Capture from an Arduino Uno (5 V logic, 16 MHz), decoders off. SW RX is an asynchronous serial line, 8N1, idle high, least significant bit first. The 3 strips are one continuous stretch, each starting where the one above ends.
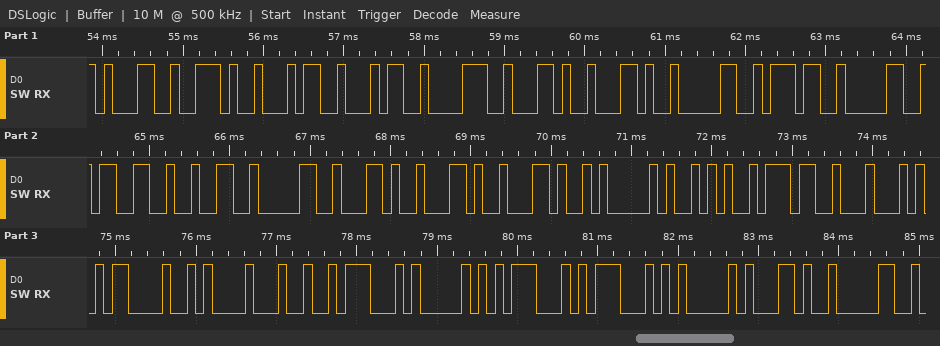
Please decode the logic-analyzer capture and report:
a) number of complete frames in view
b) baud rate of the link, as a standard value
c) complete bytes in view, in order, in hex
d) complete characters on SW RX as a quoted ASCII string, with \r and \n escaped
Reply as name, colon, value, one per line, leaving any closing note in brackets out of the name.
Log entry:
number of complete frames in view: 30
baud rate of the link, as a standard value: 9600 baud
complete bytes in view, in order, in hex: 31 2E 34 34 38 2C 2C 30 37 30 33 32 30 2C 2C 2C 41 2A 37 44 0D 0A 24 47 50 47 47 41 2C 30
complete characters on SW RX as a quoted ASCII string, with \r and \n escaped: "1.448,,070320,,,A*7D\r\n$GPGGA,0"
